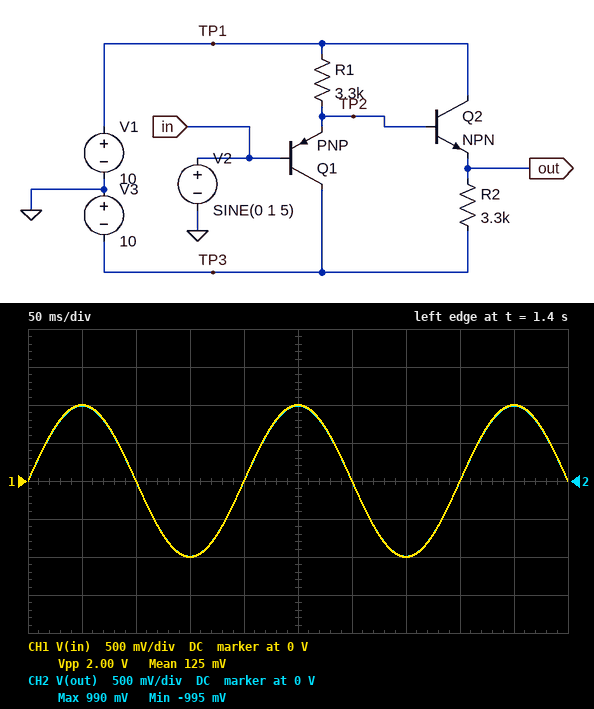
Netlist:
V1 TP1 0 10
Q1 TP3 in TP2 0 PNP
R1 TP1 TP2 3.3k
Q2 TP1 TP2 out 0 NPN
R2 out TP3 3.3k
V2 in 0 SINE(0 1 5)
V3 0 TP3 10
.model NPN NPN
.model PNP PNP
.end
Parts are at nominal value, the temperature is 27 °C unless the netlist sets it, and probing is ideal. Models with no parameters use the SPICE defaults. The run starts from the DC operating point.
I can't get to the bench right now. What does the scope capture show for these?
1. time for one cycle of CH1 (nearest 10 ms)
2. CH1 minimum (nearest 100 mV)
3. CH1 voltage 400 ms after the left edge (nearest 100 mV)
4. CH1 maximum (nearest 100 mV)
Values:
200 ms
-1.0 V
0 V
1.0 V
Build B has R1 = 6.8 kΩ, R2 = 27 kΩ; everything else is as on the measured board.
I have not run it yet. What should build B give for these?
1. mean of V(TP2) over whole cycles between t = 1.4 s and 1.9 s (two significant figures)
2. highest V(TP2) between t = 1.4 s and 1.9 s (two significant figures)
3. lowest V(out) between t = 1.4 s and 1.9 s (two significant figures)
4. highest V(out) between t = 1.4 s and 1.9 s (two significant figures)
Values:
780 mV
1.8 V
-960 mV
1.0 V
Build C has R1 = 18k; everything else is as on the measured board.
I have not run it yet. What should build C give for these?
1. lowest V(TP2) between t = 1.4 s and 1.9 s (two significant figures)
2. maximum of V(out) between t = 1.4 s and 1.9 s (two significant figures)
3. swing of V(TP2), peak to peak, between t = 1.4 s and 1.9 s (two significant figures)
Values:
-240 mV
950 mV
2.0 V
